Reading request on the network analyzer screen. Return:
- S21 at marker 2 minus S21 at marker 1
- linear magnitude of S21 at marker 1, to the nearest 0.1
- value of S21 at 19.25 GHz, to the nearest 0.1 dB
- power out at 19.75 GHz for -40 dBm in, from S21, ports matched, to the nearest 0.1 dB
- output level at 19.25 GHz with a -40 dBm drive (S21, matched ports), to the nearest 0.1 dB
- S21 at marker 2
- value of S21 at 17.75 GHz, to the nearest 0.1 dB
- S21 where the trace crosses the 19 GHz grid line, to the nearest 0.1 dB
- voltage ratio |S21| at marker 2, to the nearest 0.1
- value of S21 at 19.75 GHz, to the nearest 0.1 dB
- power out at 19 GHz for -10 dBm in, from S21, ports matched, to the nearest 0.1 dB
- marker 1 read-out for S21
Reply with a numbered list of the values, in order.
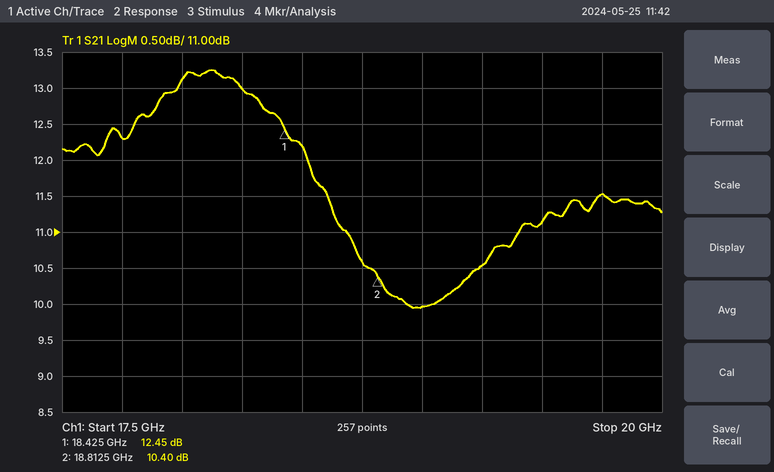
1. -2.05 dB
2. 4.2
3. 10.5 dB
4. -28.5 dBm
5. -29.5 dBm
6. 10.40 dB
7. 12.3 dB
8. 10.0 dB
9. 3.3
10. 11.5 dB
11. 0.0 dBm
12. 12.45 dB
